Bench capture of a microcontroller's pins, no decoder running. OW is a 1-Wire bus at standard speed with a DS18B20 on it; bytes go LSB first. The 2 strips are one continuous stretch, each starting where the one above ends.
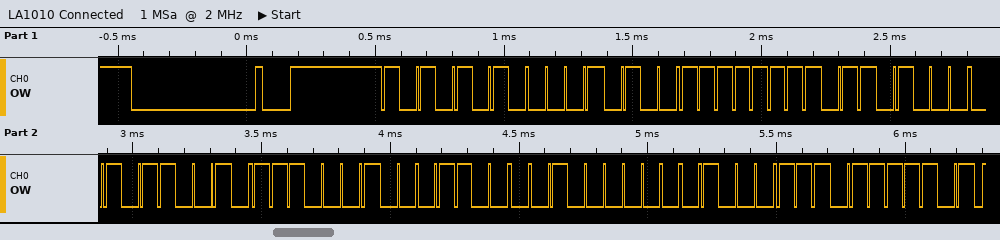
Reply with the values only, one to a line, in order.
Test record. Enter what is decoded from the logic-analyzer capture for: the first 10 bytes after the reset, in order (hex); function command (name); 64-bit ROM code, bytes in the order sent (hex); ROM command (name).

55 28 FF 16 9A 8E 18 02 E2 BE
Read Scratchpad
28 FF 16 9A 8E 18 02 E2
Match ROM
